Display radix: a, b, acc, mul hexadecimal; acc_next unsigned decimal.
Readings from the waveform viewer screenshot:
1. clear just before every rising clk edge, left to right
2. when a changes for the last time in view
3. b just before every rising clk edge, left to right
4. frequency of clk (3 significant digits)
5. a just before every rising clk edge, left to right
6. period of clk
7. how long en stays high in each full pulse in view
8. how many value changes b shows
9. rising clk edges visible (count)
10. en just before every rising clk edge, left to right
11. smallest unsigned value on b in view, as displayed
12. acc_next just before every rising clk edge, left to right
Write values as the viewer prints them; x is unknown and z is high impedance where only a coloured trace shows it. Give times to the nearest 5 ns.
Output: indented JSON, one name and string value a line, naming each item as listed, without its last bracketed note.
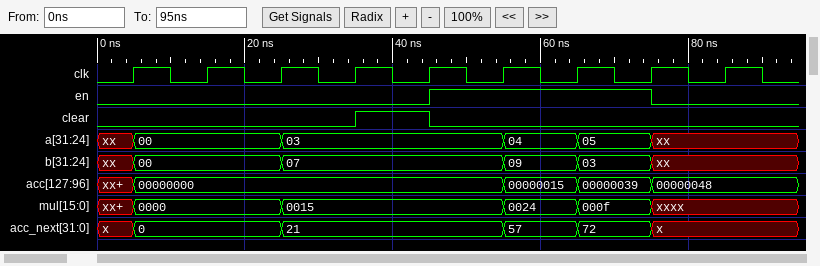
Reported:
{
  "clear just before every rising clk edge, left to right": "0 0 0 0 1 0 0 0 0",
  "when a changes for the last time in view": "75 ns",
  "b just before every rising clk edge, left to right": "xx, 00, 00, 07, 07, 07, 09, 03, xx",
  "frequency of clk": "100 MHz",
  "a just before every rising clk edge, left to right": "xx, 00, 00, 03, 03, 03, 04, 05, xx",
  "period of clk": "10 ns",
  "how long en stays high in each full pulse in view": "30 ns",
  "how many value changes b shows": "5",
  "rising clk edges visible": "9",
  "en just before every rising clk edge, left to right": "0 0 0 0 0 1 1 1 0",
  "smallest unsigned value on b in view, as displayed": "00",
  "acc_next just before every rising clk edge, left to right": "x, 0, 0, 21, 21, 21, 57, 72, x"
}
